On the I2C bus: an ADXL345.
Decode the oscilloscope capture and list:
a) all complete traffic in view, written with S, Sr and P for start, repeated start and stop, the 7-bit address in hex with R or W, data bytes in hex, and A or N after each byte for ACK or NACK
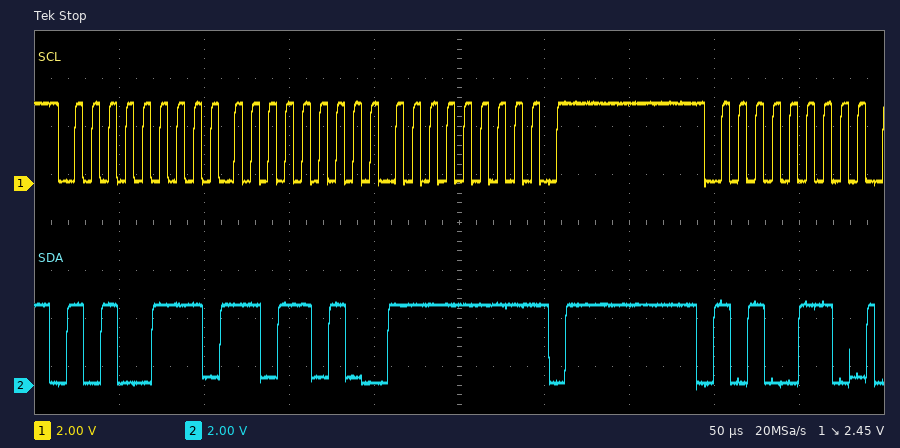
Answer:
S 53R A DA A FF N P S 53W A
